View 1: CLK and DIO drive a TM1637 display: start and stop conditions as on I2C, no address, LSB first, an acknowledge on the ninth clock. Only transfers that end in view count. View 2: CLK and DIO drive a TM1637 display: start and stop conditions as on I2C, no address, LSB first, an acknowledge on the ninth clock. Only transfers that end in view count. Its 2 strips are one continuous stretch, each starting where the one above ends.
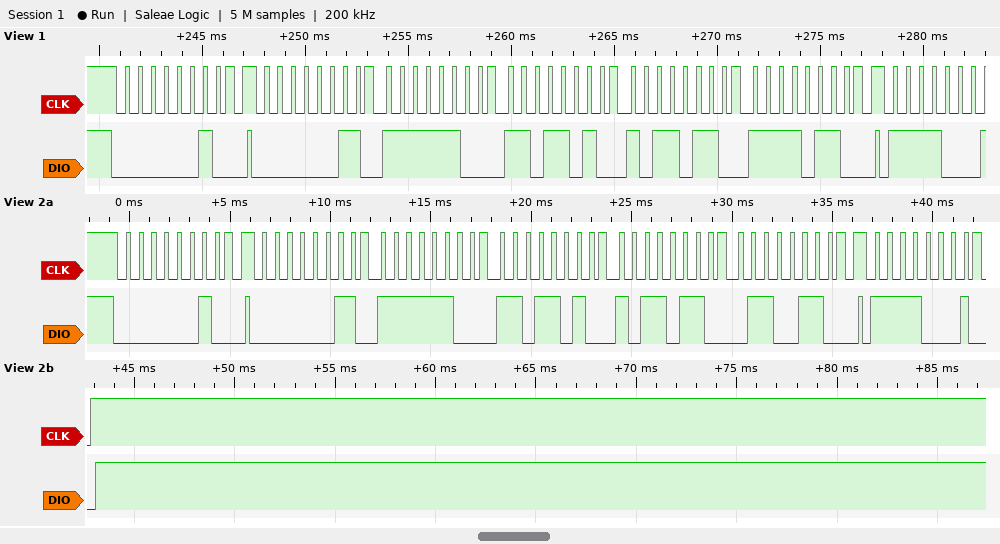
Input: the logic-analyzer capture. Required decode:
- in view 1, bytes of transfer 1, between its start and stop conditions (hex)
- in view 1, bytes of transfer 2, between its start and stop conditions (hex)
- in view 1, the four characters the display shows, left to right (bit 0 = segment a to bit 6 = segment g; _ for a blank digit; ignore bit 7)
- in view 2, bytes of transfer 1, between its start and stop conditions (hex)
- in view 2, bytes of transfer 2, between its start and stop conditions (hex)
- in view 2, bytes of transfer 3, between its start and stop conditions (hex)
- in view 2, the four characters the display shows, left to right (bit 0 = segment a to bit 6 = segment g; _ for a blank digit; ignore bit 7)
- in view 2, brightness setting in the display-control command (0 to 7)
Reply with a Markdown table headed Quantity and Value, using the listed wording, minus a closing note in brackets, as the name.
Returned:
| Quantity | Value |
|---|---|
| in view 1, bytes of transfer 1, between its start and stop conditions | 40 |
| in view 1, bytes of transfer 2, between its start and stop conditions | C0 3F 5B 6D 6F |
| in view 1, the four characters the display shows, left to right | 0259 |
| in view 2, bytes of transfer 1, between its start and stop conditions | 40 |
| in view 2, bytes of transfer 2, between its start and stop conditions | C0 3F 5B 6D 66 |
| in view 2, bytes of transfer 3, between its start and stop conditions | 8F |
| in view 2, the four characters the display shows, left to right | 0254 |
| in view 2, brightness setting in the display-control command | 7 |
